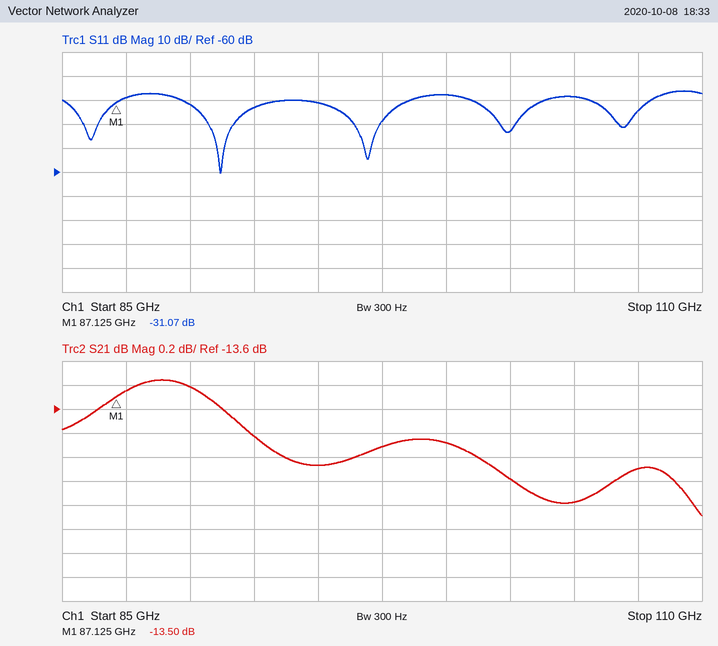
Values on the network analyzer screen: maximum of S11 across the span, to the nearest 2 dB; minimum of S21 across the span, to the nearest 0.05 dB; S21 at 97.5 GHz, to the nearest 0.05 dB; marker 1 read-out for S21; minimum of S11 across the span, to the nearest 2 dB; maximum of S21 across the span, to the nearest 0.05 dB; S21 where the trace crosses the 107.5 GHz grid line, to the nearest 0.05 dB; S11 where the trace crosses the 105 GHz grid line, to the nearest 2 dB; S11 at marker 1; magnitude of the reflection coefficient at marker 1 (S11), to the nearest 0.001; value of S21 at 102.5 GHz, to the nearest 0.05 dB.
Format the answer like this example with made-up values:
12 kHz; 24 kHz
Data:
-26 dB; -14.50 dB; -13.90 dB; -13.50 dB; -60 dB; -13.35 dB; -14.10 dB; -28 dB; -31.07 dB; 0.028; -14.20 dB
